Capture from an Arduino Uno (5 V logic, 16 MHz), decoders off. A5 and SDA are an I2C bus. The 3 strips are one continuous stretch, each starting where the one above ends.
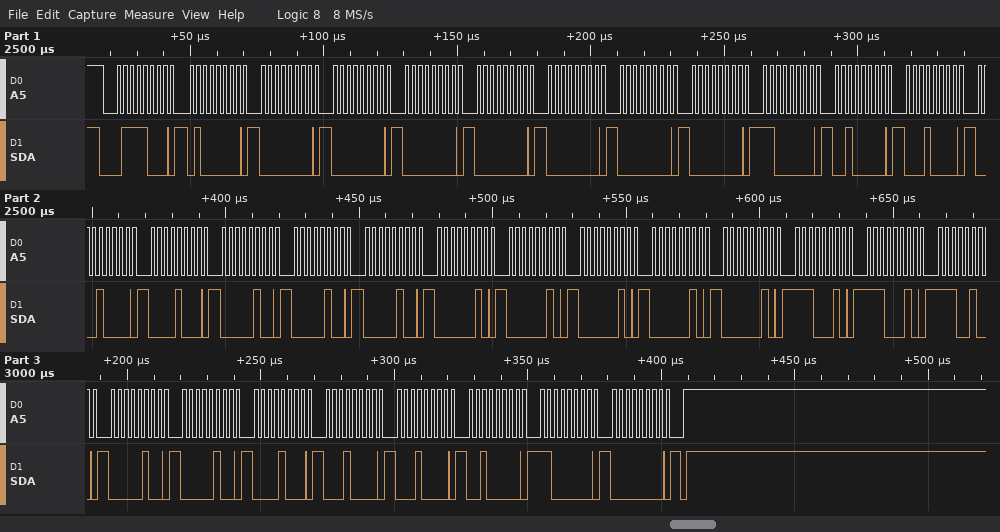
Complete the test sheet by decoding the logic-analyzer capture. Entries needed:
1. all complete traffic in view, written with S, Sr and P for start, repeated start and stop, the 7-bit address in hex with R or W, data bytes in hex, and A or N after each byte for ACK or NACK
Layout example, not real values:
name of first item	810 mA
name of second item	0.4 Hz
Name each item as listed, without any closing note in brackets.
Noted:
all complete traffic in view, written with S, Sr and P for start, repeated start and stop, the 7-bit address in hex with R or W, data bytes in hex, and A or N after each byte for ACK or NACK	S 3CW A 40 A 00 A 00 A 00 A 00 A 00 A 00 A 00 A C0 A 20 A 10 A 10 A 08 A 04 A 04 A 04 A 02 A 02 A 02 A 02 A 02 A E2 A E2 A E4 A 04 A 04 A 08 A 10 A 10 A 20 A C0 A 00 A P
